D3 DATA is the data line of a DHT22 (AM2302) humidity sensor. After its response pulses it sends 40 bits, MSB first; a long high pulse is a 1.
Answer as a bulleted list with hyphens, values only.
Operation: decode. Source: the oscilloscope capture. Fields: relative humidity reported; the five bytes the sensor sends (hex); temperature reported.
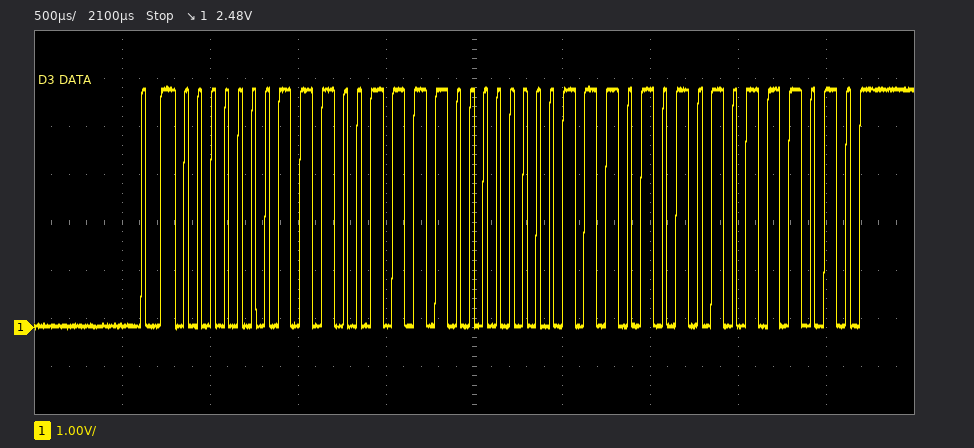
- 46.3 %
- 01 CF 00 EA BA
- 23.4 °C
